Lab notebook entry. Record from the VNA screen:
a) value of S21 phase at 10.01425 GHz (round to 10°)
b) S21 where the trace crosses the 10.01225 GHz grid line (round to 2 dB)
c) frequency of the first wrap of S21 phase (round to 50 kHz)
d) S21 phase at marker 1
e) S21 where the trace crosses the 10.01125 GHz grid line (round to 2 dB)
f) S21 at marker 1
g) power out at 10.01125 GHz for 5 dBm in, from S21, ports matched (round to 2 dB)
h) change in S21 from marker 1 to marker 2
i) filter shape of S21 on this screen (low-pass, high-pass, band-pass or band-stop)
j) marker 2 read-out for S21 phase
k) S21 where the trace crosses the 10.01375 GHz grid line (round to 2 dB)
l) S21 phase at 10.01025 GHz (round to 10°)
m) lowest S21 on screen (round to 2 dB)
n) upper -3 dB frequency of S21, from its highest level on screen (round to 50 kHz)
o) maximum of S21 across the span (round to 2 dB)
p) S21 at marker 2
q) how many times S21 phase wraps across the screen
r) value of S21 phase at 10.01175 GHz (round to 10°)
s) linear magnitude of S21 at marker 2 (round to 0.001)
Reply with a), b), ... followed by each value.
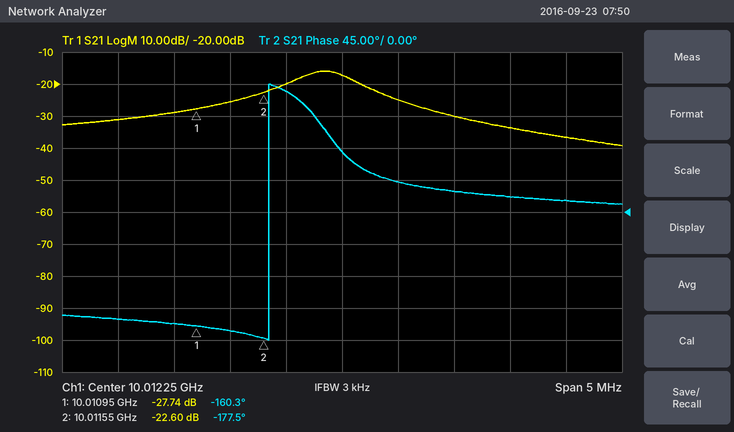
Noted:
a) 20°
b) -18 dB
c) 10.01160 GHz
d) -160.3°
e) -26 dB
f) -27.74 dB
g) -20 dBm
h) 5.14 dB
i) band-pass
j) -177.5°
k) -34 dB
l) -150°
m) -40 dB
n) 10.01235 GHz
o) -16 dB
p) -22.60 dB
q) 1
r) 170°
s) 0.074
